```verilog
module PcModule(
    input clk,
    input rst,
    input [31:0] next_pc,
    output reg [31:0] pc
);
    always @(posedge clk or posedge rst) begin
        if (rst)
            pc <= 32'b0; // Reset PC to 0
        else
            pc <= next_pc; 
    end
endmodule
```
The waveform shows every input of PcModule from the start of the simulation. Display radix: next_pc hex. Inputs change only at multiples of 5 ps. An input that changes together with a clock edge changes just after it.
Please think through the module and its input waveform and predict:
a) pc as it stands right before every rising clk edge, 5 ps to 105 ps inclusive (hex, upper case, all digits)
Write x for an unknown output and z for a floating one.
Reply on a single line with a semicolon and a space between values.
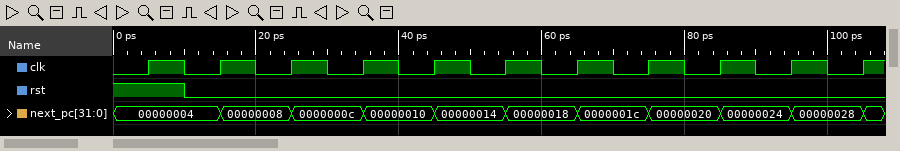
00000000, 00000000, 00000004, 00000008, 0000000C, 00000010, 00000014, 00000018, 0000001C, 00000020, 00000024
